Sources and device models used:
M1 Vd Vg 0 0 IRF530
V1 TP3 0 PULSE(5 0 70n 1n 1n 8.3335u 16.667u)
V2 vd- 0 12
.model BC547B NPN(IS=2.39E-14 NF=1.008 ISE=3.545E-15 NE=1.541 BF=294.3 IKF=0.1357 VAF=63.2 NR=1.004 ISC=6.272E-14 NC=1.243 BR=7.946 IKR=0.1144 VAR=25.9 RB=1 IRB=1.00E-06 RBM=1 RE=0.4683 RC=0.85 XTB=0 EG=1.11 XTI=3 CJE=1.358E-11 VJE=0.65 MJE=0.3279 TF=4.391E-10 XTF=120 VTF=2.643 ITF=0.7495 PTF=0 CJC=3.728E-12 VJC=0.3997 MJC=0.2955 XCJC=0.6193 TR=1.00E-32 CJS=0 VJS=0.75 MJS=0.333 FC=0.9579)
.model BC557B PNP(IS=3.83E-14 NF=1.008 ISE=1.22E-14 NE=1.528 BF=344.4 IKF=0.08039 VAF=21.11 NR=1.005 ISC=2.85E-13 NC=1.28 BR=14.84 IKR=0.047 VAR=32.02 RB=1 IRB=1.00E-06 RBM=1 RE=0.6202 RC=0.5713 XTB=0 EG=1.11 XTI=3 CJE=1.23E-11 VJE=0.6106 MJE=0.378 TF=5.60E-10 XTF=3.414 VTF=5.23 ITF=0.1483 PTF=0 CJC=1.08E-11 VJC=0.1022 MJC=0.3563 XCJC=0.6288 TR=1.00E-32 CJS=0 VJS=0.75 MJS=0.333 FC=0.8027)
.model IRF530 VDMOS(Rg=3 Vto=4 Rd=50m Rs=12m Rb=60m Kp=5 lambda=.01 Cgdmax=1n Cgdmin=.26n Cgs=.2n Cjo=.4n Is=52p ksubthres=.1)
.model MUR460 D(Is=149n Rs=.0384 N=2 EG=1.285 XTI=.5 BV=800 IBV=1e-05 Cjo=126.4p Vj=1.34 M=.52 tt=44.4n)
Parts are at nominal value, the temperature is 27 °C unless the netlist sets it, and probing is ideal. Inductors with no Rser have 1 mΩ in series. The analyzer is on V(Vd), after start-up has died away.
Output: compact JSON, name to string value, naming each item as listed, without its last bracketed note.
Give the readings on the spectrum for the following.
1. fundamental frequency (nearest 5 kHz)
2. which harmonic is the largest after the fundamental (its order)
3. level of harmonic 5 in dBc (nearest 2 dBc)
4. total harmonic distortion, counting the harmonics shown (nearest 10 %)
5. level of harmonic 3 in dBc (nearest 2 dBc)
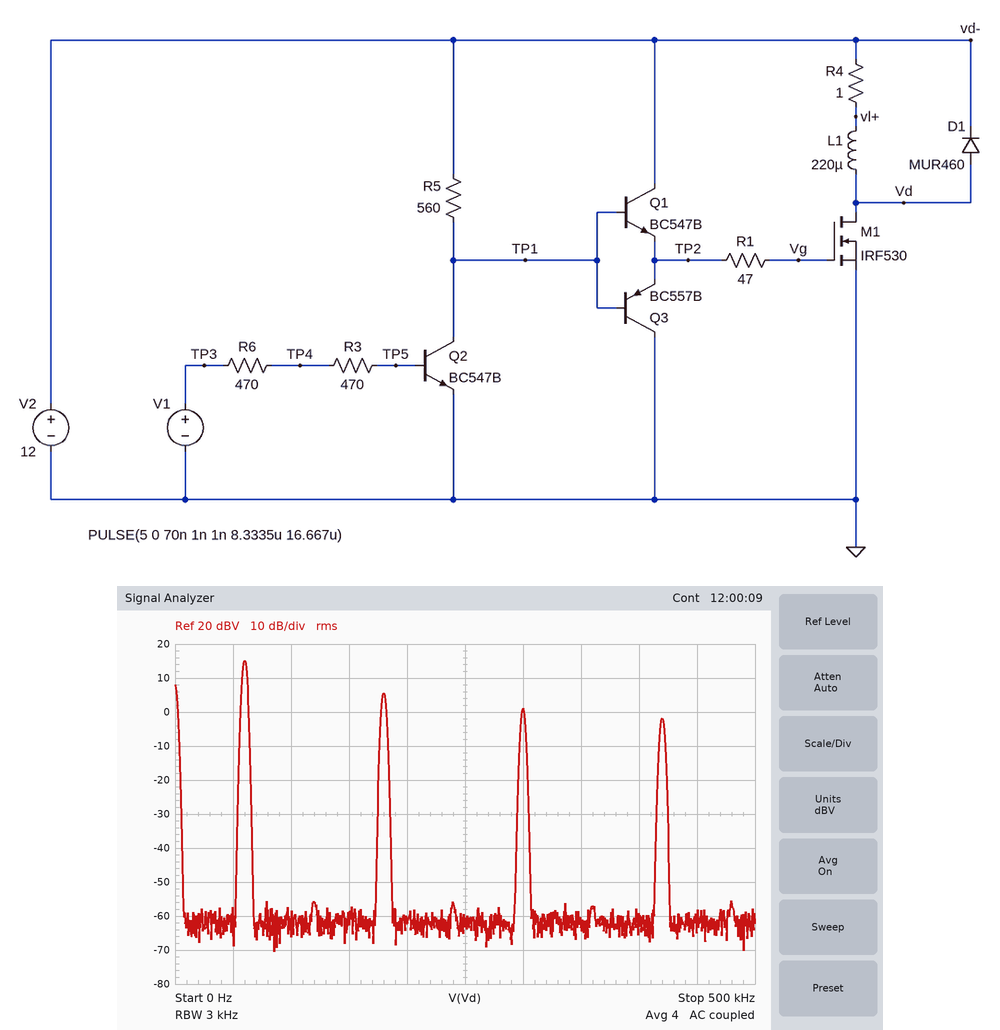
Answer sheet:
{"fundamental frequency": "60 kHz", "which harmonic is the largest after the fundamental": "3", "level of harmonic 5 in dBc": "-14 dBc", "total harmonic distortion, counting the harmonics shown": "40 %", "level of harmonic 3 in dBc": "-10 dBc"}
